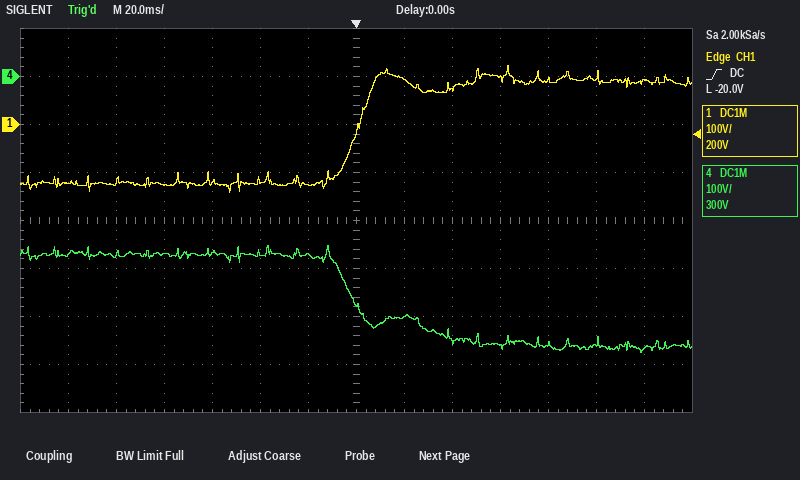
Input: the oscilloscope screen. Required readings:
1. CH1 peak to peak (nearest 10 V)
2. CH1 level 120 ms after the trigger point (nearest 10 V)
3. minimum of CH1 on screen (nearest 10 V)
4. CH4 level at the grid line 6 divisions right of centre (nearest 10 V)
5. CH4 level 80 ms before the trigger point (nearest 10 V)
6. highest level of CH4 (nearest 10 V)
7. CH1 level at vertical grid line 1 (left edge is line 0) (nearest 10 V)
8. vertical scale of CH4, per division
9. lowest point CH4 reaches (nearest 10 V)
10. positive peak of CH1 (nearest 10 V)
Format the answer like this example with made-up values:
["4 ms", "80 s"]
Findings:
["260 V", "90 V", "-140 V", "-570 V", "-370 V", "-350 V", "-120 V", "100 V", "-580 V", "120 V"]
